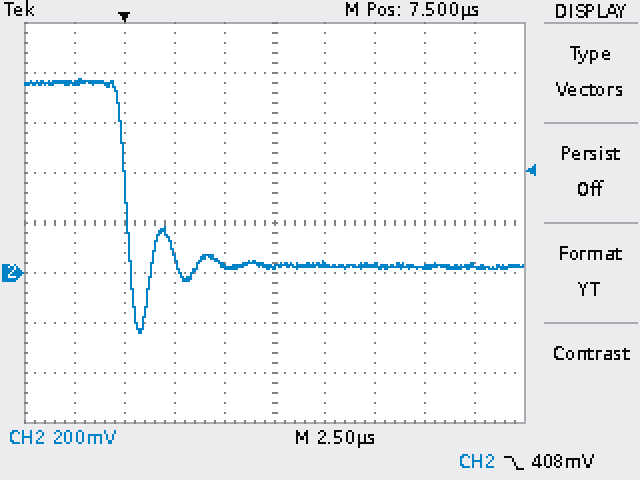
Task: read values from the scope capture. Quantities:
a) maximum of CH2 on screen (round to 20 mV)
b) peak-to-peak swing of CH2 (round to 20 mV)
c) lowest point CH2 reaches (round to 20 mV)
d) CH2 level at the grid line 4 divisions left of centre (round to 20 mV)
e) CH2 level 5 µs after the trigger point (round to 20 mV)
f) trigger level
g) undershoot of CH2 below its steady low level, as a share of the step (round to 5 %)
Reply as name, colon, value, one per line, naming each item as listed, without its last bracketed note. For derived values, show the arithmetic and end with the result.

maximum of CH2 on screen: 780 mV
peak-to-peak swing of CH2: 780 mV − (-240 mV) = 1.02 V
lowest point CH2 reaches: -240 mV
CH2 level at the grid line 4 divisions left of centre: 760 mV
CH2 level 5 µs after the trigger point: 20 mV
trigger level: 408 mV
undershoot of CH2 below its steady low level, as a share of the step: 35 %
